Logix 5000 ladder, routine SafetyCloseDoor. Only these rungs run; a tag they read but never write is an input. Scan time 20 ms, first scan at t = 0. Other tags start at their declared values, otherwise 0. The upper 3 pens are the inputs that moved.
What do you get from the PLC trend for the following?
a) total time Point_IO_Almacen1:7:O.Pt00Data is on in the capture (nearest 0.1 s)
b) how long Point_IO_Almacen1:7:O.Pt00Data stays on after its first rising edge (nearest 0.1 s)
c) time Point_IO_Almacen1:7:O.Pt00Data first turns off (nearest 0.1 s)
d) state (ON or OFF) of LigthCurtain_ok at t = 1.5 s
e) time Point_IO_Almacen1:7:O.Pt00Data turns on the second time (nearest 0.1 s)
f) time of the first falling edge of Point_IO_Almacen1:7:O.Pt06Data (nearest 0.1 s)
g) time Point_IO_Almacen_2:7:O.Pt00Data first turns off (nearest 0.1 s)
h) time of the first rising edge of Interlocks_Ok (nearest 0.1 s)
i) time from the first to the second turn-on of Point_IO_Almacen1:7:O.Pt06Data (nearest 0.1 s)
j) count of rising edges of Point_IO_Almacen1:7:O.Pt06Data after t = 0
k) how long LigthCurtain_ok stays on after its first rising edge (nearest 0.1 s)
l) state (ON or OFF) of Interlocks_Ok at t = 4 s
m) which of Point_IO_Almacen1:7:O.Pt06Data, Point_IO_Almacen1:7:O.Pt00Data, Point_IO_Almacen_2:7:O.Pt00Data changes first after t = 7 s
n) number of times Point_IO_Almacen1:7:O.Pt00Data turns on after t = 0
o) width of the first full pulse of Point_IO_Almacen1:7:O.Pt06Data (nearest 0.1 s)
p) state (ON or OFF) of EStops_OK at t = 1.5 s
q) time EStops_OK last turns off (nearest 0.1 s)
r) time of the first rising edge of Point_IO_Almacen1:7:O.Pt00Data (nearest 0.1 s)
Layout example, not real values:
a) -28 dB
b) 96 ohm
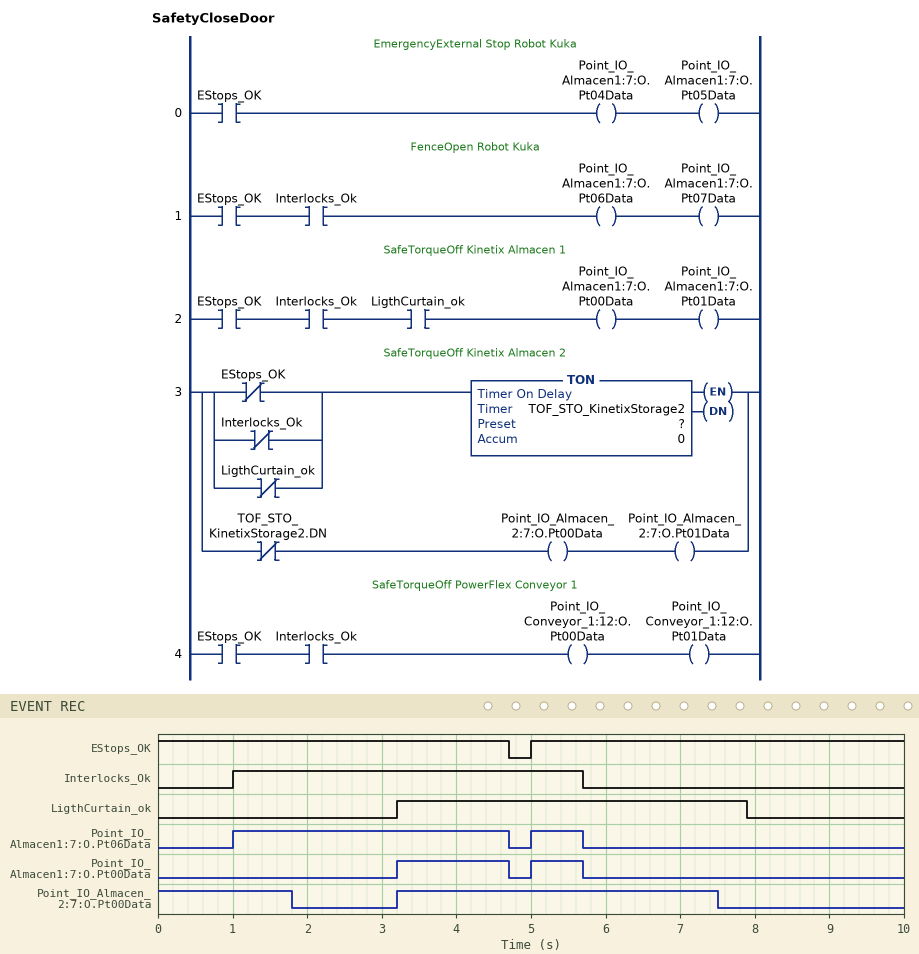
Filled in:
a) 2.2 s
b) 1.5 s
c) 4.7 s
d) OFF
e) 5.0 s
f) 4.7 s
g) 1.8 s
h) 1.0 s
i) 4.0 s
j) 2
k) 4.7 s
l) ON
m) Point_IO_Almacen_2:7:O.Pt00Data
n) 2
o) 3.7 s
p) ON
q) 4.7 s
r) 3.2 s
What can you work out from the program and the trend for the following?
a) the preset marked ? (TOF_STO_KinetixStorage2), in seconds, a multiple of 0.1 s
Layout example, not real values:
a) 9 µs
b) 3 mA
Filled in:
a) 1.8 s
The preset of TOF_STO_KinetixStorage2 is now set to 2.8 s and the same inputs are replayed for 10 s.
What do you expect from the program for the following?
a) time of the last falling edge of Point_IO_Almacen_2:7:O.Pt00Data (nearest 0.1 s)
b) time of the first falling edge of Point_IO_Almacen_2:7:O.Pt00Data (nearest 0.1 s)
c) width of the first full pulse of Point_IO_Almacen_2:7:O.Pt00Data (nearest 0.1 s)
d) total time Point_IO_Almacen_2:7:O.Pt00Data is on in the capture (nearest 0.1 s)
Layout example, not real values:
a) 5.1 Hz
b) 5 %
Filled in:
a) 8.5 s
b) 2.8 s
c) 5.3 s
d) 8.1 s
